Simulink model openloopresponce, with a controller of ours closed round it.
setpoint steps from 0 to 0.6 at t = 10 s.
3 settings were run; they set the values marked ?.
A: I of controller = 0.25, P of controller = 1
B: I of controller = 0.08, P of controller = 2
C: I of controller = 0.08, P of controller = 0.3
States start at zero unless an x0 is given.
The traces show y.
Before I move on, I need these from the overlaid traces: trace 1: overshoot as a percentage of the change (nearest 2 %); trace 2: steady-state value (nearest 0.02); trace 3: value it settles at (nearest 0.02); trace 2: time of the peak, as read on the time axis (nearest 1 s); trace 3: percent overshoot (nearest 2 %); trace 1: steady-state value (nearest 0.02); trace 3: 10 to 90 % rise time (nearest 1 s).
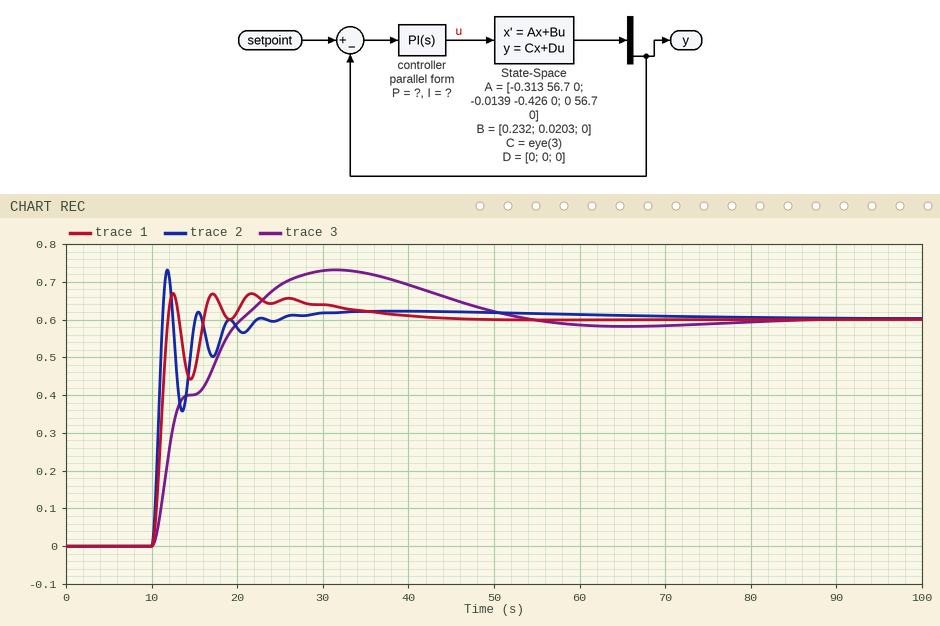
12 %
0.60
0.60
12 s
22 %
0.60
8 s
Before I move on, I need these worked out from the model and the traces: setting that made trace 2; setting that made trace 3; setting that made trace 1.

B
C
A
